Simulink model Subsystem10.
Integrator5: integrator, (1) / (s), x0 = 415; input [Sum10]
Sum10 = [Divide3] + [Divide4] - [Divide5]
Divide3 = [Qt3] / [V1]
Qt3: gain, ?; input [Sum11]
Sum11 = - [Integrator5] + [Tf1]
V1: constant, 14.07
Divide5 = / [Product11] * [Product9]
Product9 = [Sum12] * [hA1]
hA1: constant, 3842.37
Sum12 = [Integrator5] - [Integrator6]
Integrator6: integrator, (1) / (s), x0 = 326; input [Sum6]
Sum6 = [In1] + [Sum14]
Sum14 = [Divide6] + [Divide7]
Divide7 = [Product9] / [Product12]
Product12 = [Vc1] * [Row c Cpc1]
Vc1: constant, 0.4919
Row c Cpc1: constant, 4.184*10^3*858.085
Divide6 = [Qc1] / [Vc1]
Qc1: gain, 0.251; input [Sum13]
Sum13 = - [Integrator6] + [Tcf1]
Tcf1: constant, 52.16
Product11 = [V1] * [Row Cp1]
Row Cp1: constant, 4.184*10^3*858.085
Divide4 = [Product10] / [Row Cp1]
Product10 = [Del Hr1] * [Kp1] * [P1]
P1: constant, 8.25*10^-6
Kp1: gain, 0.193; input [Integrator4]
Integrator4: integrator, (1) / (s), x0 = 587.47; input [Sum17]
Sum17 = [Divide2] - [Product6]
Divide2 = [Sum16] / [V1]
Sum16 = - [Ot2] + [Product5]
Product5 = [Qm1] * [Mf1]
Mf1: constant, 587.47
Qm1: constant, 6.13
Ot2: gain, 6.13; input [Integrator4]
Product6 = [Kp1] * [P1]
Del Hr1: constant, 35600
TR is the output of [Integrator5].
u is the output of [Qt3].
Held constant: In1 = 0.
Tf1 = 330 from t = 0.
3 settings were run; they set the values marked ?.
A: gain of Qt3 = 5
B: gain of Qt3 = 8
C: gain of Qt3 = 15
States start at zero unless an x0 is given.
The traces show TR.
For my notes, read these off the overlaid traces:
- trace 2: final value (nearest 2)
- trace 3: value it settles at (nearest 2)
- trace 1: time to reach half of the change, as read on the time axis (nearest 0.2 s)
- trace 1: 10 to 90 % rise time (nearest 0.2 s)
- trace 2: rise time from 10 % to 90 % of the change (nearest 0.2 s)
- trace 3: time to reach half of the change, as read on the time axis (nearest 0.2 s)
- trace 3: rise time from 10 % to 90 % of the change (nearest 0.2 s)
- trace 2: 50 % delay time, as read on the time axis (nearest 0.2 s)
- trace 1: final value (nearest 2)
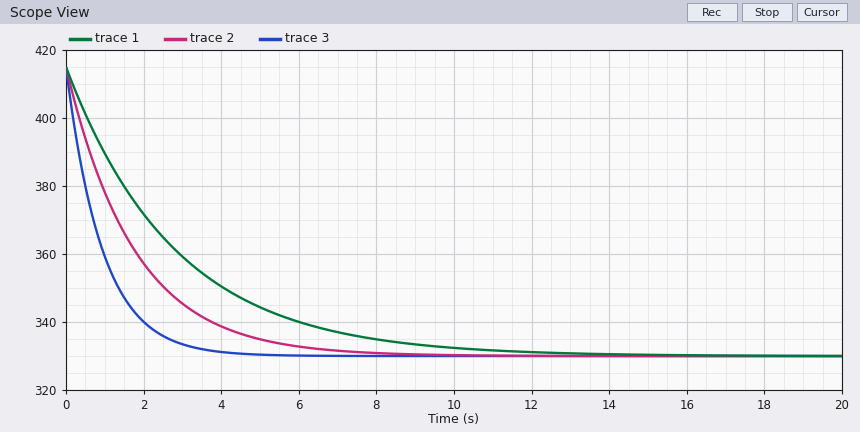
330
330
2.0 s
6.2 s
3.8 s
0.6 s
2.0 s
1.2 s
330
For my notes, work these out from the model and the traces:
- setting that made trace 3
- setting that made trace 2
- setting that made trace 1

C
B
A
